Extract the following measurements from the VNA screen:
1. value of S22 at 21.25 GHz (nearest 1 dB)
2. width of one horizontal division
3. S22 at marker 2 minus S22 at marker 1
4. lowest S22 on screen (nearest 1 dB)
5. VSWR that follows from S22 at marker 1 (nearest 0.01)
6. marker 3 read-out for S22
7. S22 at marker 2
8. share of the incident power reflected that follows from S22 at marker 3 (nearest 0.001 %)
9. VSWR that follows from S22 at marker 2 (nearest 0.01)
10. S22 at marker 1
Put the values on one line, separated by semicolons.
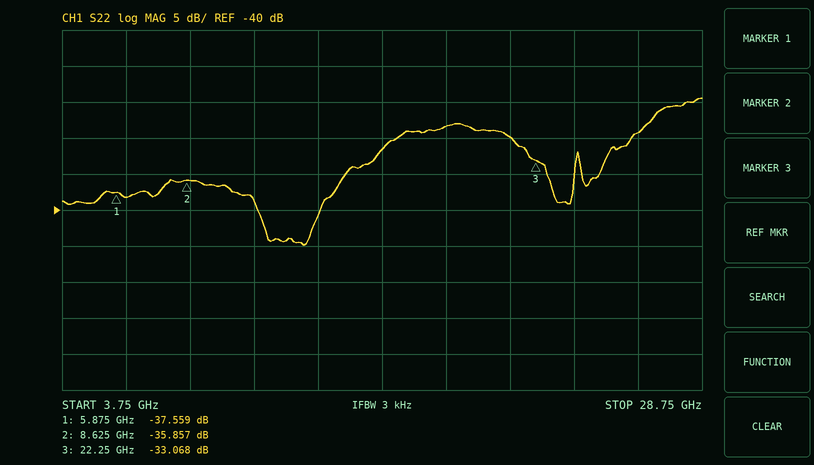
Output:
-30 dB; 2.5 GHz; 1.702 dB; -45 dB; 1.03; -33.068 dB; -35.857 dB; 0.049 %; 1.03; -37.559 dB
